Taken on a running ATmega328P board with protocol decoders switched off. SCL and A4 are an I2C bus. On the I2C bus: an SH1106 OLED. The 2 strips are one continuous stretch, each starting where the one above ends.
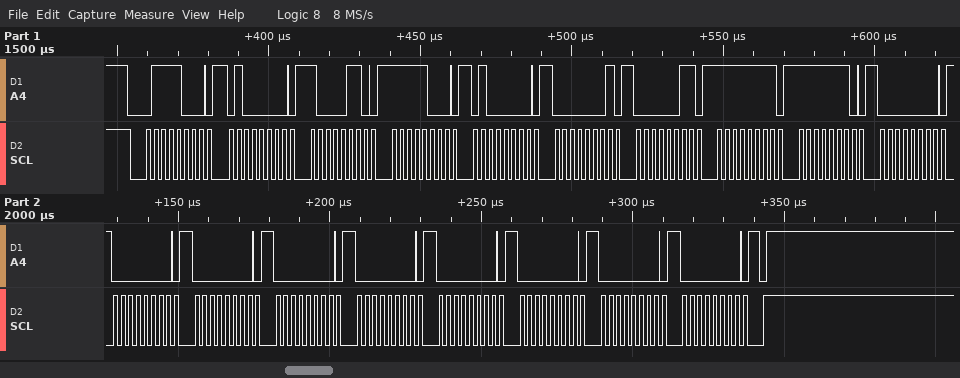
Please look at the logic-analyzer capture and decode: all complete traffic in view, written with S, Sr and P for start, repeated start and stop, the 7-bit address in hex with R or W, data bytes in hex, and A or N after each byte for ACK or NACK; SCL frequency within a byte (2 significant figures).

S 3CW A 40 A 86 A F8 A 40 A 01 A 03 A FF A FE A 00 A 00 A 00 A 00 A 00 A 00 A 00 A 00 A 00 A P
400 kHz
